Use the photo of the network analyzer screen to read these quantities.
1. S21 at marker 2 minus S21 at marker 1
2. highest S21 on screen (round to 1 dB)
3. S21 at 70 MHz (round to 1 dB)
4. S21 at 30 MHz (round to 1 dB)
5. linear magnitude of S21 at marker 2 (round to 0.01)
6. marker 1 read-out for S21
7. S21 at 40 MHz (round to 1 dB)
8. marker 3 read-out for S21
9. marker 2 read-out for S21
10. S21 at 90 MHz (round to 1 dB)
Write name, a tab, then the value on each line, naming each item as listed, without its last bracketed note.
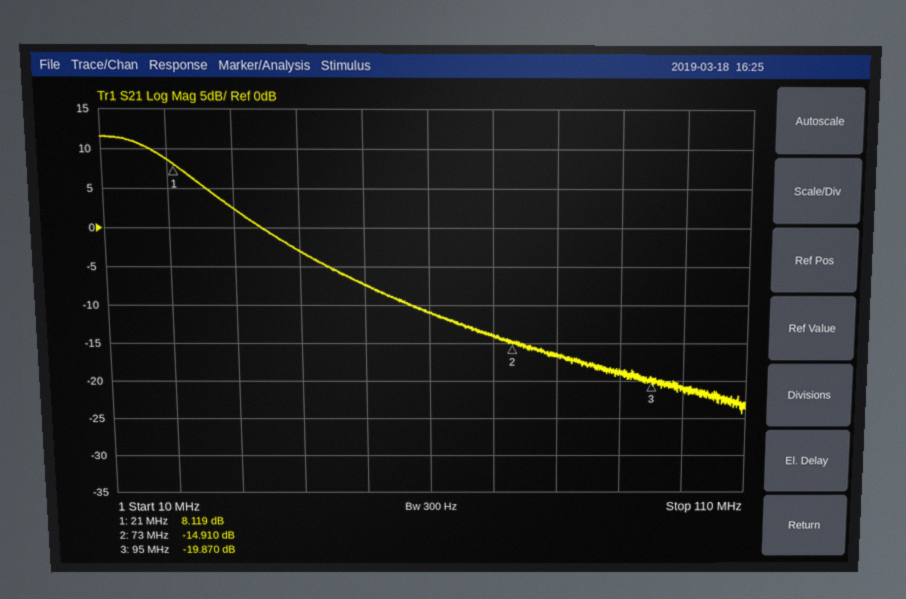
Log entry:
S21 at marker 2 minus S21 at marker 1	-23.029 dB
highest S21 on screen	12 dB
S21 at 70 MHz	-14 dB
S21 at 30 MHz	2 dB
linear magnitude of S21 at marker 2	0.18
marker 1 read-out for S21	8.119 dB
S21 at 40 MHz	-3 dB
marker 3 read-out for S21	-19.870 dB
marker 2 read-out for S21	-14.910 dB
S21 at 90 MHz	-19 dB
